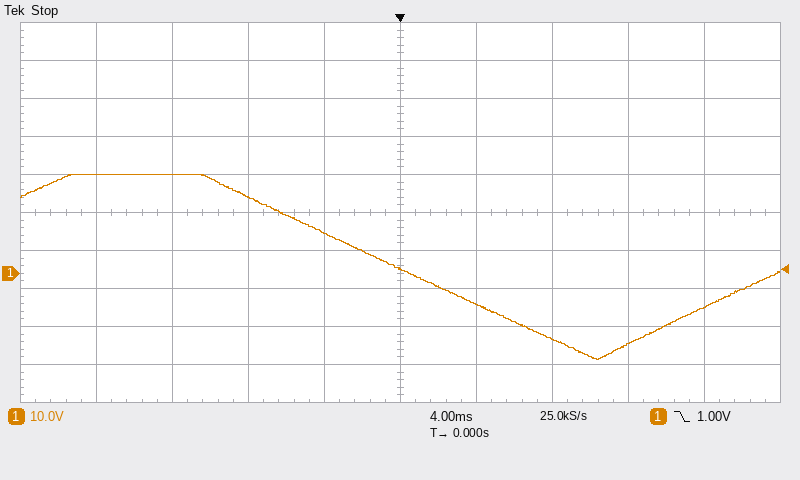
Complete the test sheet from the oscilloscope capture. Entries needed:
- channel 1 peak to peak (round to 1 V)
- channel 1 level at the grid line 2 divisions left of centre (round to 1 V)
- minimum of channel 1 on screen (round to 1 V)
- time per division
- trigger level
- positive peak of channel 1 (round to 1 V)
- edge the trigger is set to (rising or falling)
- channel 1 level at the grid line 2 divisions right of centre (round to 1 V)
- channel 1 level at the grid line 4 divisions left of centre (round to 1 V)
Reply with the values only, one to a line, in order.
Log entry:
49 V
20 V
-23 V
4 ms
1.00 V
26 V
falling
-17 V
26 V
